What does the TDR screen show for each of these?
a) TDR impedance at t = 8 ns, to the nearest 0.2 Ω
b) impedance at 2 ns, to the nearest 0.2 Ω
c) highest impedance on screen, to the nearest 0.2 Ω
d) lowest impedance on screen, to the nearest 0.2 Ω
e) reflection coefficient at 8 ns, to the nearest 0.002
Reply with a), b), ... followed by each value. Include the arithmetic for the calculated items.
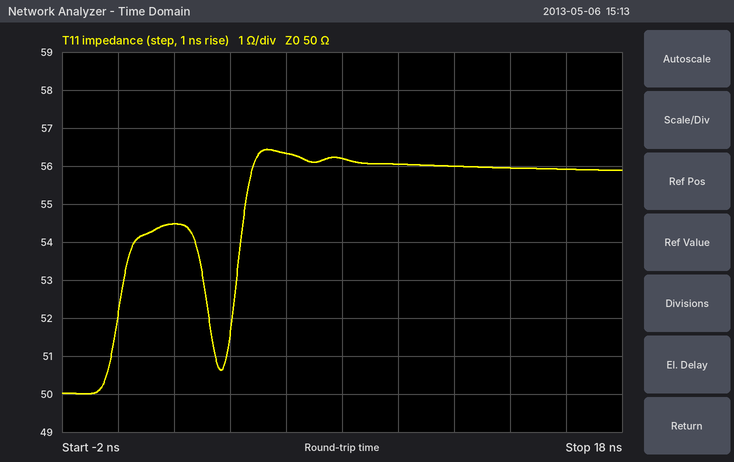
a) 56.2 Ω
b) 54.4 Ω
c) 56.4 Ω
d) 50.0 Ω
e) (56.2 − 50)/(56.2 + 50) ≈ +0.058
